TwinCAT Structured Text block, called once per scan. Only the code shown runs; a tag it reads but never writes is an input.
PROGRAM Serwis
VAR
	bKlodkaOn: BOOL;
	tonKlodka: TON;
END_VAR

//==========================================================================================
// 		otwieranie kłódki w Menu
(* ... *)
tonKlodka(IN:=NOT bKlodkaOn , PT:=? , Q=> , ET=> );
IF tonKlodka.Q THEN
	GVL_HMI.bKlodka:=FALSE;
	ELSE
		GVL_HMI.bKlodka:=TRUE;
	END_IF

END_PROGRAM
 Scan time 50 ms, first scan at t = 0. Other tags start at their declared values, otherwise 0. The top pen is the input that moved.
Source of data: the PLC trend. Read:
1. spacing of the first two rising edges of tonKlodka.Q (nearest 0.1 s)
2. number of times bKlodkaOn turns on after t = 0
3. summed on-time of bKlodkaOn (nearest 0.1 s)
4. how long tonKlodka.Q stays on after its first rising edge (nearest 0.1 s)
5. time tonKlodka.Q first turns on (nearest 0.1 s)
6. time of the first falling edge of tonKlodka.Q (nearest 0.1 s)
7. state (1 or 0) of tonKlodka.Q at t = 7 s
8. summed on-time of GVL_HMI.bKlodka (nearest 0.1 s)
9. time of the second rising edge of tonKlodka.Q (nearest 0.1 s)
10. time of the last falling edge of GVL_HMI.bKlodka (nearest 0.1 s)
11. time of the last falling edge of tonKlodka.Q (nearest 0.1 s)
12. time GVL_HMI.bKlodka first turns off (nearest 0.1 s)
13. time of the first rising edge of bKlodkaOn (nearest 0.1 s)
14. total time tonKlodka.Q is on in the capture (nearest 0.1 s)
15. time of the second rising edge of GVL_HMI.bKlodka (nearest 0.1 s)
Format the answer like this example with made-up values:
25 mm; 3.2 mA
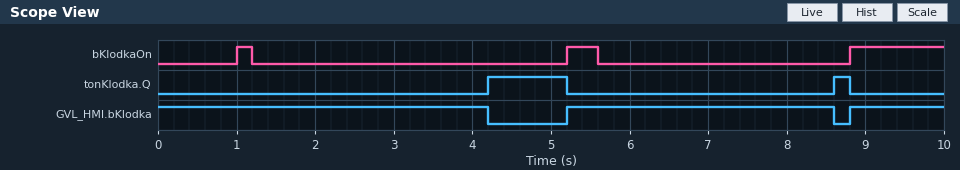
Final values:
4.4 s; 3; 1.8 s; 1.0 s; 4.2 s; 5.2 s; 0; 8.8 s; 8.6 s; 8.6 s; 8.8 s; 4.2 s; 1.0 s; 1.2 s; 8.8 s
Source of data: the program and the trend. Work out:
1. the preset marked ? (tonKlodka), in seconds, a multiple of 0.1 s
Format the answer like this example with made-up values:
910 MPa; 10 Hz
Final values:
3.0 s
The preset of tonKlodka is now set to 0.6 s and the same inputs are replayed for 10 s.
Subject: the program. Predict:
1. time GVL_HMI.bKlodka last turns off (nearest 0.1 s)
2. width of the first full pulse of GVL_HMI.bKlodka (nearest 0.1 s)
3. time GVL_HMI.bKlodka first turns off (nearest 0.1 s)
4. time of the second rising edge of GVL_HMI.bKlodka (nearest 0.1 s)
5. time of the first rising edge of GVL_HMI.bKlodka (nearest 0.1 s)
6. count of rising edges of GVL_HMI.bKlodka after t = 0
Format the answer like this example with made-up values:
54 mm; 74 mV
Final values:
6.2 s; 0.8 s; 0.6 s; 5.2 s; 1.0 s; 3
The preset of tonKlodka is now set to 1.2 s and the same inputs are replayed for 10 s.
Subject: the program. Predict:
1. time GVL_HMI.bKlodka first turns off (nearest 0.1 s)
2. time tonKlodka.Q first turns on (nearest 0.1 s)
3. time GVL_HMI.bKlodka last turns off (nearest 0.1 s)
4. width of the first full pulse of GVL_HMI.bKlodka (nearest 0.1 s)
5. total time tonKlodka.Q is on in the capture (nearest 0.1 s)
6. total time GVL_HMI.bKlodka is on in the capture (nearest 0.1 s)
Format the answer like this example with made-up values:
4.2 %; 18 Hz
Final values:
2.4 s; 2.4 s; 6.8 s; 1.6 s; 4.8 s; 5.2 s
